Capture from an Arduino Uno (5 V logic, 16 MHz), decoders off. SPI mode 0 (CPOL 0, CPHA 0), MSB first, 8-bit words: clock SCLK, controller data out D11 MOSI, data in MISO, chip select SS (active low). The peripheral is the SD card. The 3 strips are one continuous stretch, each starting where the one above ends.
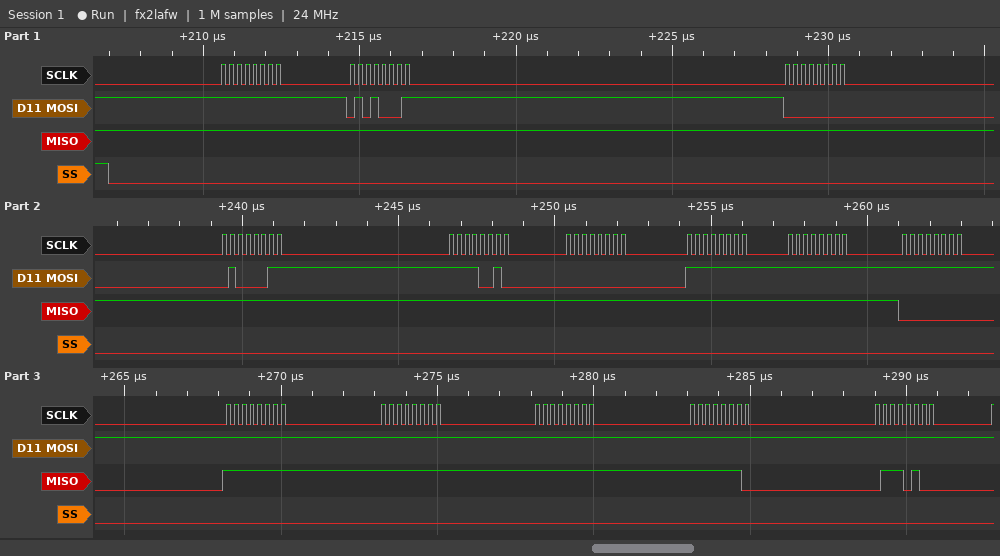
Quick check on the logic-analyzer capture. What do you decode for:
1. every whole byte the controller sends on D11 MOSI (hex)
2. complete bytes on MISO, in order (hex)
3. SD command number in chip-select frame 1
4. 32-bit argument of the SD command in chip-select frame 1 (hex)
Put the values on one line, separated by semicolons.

0xFF 0x51 0x00 0x43 0xF2 0x00 0xFF 0xFF 0xFF 0xFF 0xFF 0xFF 0xFF 0xFF; 0xFF 0xFF 0xFF 0xFF 0xFF 0xFF 0xFF 0xFF 0x00 0xFF 0xFF 0xFF 0xFE 0x74; CMD17; 0x0043F200
